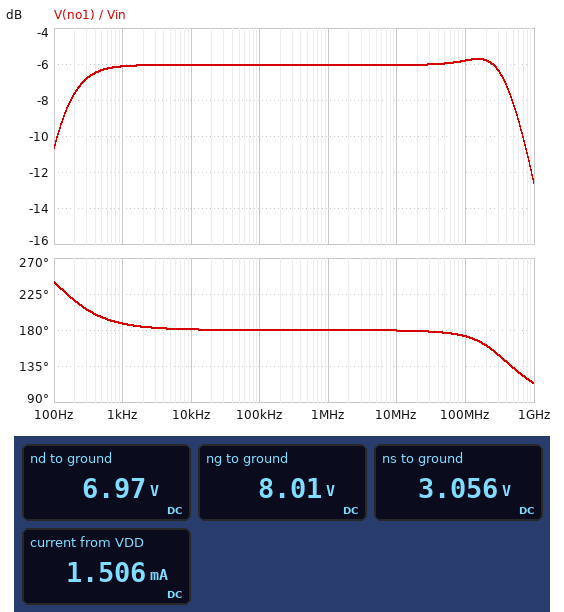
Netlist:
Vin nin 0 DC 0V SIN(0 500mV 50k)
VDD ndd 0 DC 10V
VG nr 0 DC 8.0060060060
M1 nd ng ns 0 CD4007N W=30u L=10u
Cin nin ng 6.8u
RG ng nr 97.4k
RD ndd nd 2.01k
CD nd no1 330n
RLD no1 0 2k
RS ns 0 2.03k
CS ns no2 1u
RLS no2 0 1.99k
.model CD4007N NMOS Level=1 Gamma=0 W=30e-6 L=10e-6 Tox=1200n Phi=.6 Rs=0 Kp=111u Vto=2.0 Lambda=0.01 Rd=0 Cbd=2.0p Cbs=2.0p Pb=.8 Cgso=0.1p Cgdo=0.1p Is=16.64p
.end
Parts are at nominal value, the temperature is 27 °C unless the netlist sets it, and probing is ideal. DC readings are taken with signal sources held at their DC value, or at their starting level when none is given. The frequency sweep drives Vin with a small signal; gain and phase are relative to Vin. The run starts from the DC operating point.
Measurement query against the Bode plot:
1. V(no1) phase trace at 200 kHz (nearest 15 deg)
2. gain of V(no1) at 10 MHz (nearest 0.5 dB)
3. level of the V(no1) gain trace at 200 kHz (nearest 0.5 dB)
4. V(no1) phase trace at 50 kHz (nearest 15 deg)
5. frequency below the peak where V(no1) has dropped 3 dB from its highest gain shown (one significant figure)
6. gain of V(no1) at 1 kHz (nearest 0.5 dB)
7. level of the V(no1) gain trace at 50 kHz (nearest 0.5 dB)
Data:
180 deg
-6.0 dB
-6.0 dB
180 deg
100 Hz
-6.0 dB
-6.0 dB
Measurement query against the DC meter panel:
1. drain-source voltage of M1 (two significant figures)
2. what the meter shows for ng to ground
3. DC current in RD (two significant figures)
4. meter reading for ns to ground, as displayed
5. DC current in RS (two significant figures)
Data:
3.9 V
8.01 V
1.5 mA
3.056 V
1.5 mA
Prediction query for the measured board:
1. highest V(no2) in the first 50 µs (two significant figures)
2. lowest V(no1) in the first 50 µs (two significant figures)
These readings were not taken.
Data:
250 mV
-250 mV
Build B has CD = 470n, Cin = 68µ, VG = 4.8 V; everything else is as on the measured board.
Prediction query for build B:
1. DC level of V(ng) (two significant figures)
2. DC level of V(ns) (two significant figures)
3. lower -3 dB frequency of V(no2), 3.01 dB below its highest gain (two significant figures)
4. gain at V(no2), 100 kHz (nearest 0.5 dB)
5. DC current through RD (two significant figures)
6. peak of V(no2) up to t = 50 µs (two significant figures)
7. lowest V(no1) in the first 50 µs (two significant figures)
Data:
4.8 V
1.1 V
55 Hz
-8.5 dB
530 µA
200 mV
-200 mV
